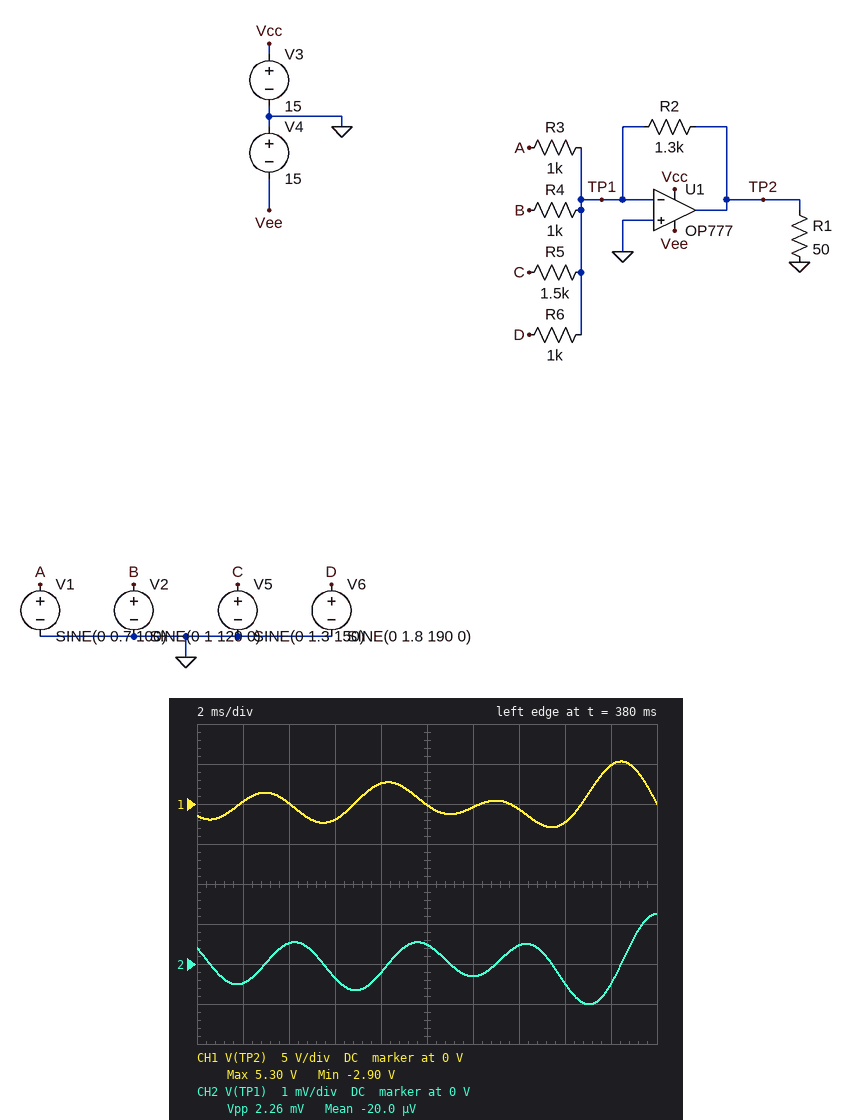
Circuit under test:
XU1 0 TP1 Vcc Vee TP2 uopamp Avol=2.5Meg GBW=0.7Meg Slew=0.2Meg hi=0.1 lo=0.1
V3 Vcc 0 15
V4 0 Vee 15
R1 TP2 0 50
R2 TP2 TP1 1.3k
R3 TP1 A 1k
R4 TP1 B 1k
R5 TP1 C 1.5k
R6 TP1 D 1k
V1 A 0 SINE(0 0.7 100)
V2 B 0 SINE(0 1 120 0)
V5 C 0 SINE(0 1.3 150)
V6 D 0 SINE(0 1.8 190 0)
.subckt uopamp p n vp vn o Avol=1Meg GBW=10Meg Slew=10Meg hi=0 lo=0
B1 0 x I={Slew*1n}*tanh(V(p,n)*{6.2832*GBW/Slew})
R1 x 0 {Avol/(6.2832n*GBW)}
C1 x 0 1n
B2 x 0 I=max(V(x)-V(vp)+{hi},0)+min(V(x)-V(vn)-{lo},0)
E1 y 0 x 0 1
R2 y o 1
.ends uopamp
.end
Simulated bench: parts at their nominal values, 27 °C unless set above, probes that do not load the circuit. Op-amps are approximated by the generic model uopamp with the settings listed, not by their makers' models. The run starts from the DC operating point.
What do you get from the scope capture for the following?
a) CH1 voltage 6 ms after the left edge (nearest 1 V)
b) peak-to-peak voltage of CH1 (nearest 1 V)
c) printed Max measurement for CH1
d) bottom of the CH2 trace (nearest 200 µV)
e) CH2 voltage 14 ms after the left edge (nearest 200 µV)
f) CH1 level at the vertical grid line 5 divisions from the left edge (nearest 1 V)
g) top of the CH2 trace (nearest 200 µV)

-2 V
8 V
5.30 V
-1.0 mV
400 µV
0 V
1.2 mV
